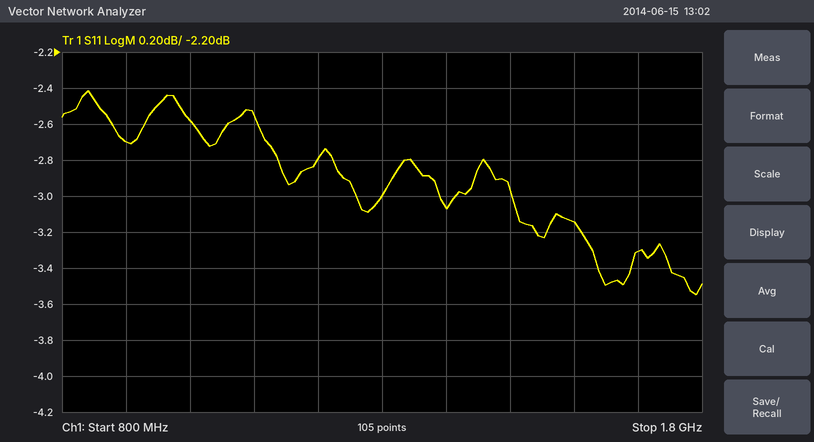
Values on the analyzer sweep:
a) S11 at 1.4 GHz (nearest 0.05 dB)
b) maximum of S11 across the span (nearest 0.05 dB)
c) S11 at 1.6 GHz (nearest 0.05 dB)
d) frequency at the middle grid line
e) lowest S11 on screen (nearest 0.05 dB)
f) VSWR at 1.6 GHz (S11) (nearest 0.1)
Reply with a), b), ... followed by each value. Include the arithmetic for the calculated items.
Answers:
a) -3.05 dB
b) -2.40 dB
c) -3.15 dB
d) 1.3 GHz
e) -3.55 dB
f) |Γ| = 10^(-3.15/20) = 0.6958; VSWR = (1 + 0.6958)/(1 − 0.6958) ≈ 5.6
